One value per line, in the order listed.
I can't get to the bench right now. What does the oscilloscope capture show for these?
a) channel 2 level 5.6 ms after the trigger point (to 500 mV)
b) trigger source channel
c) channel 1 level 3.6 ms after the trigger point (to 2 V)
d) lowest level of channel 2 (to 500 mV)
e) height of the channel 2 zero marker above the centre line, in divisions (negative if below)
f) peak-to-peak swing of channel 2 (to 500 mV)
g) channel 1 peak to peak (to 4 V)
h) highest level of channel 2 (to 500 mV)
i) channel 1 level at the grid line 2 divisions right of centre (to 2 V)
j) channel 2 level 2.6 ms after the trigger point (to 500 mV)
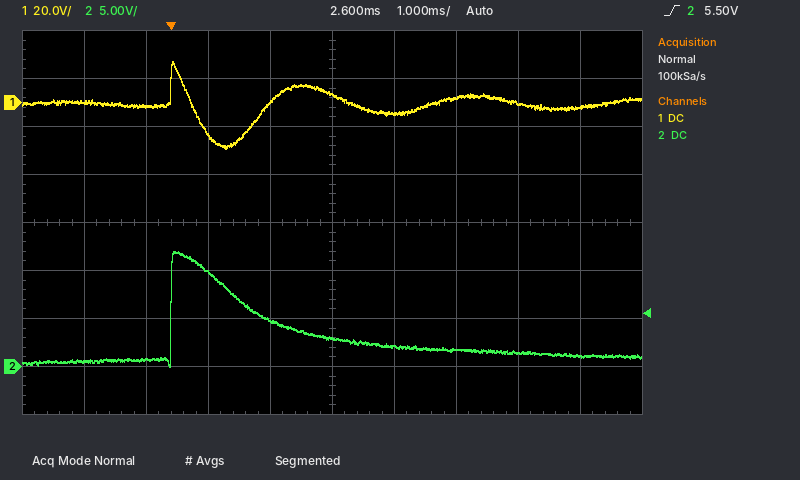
1.5 V
channel 2
-4 V
0.0 V
-3.0 div
12.0 V
36 V
12.0 V
2 V
3.0 V
